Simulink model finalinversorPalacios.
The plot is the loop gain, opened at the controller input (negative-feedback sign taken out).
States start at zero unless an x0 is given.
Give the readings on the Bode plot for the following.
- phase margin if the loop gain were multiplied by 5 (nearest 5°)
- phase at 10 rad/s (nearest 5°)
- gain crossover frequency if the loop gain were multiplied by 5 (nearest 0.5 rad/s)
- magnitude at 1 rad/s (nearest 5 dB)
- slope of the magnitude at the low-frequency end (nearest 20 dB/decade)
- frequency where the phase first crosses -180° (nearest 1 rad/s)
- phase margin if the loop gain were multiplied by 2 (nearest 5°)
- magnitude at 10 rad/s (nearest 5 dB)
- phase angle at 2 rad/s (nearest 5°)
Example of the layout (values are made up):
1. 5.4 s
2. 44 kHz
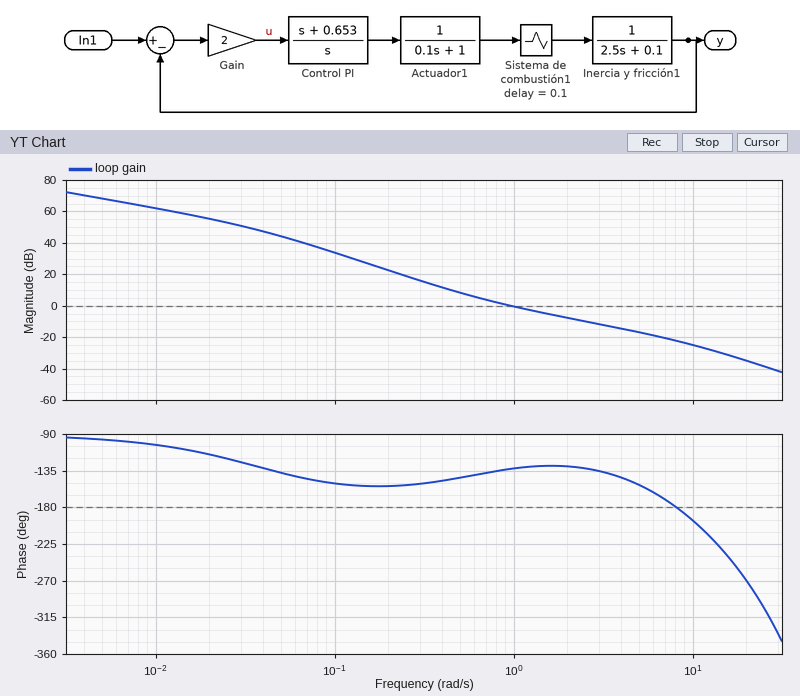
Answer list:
1. 40°
2. -195°
3. 4.0 rad/s
4. 0 dB
5. -20 dB/decade
6. 8 rad/s
7. 50°
8. -25 dB
9. -130°
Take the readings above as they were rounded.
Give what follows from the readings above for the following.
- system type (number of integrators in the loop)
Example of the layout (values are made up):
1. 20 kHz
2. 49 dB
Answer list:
1. 1
